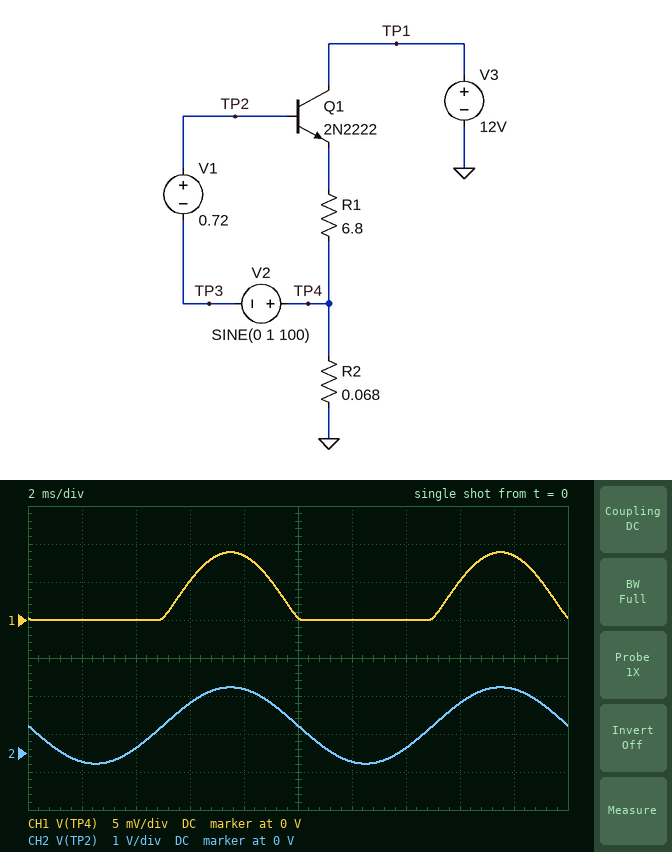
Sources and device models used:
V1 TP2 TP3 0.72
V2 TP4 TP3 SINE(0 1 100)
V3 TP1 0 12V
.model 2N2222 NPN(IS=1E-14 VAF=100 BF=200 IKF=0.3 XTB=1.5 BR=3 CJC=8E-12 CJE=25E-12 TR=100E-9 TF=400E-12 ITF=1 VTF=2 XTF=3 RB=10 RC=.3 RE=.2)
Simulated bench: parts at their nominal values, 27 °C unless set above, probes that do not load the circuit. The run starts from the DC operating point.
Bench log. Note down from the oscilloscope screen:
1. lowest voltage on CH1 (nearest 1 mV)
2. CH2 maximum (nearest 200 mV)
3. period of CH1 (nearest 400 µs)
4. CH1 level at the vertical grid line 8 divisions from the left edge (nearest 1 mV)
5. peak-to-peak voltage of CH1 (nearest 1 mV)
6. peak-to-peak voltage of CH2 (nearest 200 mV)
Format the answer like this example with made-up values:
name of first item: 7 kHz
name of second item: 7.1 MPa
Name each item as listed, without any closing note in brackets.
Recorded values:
lowest voltage on CH1: 0 V
CH2 maximum: 1.8 V
period of CH1: 10.0 ms
CH1 level at the vertical grid line 8 divisions from the left edge: 5 mV
peak-to-peak voltage of CH1: 9 mV
peak-to-peak voltage of CH2: 2.0 V
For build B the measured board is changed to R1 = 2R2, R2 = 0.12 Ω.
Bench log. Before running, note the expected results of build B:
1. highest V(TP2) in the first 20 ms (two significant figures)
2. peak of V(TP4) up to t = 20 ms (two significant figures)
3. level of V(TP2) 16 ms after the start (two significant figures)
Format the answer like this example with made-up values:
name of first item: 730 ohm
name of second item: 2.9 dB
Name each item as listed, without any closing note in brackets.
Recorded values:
highest V(TP2) in the first 20 ms: 1.8 V
peak of V(TP4) up to t = 20 ms: 43 mV
level of V(TP2) 16 ms after the start: 1.3 V
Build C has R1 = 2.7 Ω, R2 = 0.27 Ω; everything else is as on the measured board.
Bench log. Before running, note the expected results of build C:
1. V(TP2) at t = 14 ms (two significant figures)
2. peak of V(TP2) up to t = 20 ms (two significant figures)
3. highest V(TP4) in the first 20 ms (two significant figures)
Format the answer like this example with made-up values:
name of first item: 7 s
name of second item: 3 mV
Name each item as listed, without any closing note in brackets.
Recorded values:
V(TP2) at t = 14 ms: 130 mV
peak of V(TP2) up to t = 20 ms: 1.8 V
highest V(TP4) in the first 20 ms: 81 mV
